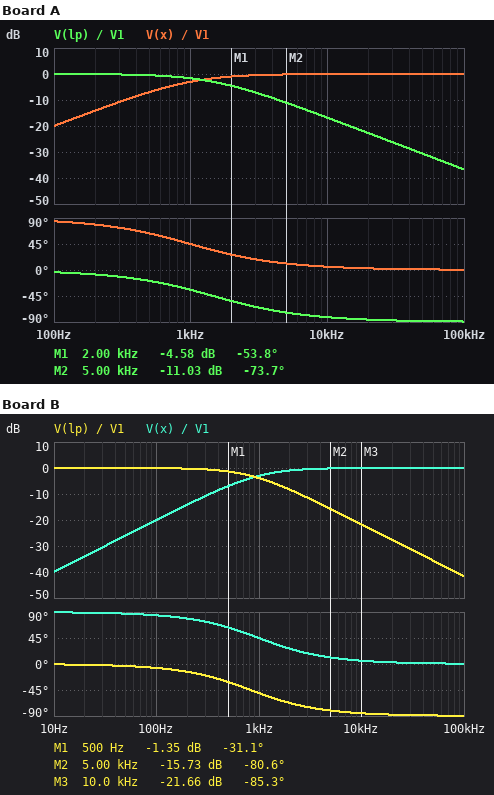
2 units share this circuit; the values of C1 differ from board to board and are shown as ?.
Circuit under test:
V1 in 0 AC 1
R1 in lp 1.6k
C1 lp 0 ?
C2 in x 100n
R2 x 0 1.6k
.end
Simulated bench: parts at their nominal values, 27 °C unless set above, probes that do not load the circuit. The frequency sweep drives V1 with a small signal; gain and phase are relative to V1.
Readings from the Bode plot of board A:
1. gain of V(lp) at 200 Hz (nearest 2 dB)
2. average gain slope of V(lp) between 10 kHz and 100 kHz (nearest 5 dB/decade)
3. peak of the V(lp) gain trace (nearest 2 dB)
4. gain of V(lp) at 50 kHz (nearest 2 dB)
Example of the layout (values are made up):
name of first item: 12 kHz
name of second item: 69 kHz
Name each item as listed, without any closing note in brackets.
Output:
gain of V(lp) at 200 Hz: 0 dB
average gain slope of V(lp) between 10 kHz and 100 kHz: -20 dB/decade
peak of the V(lp) gain trace: 0 dB
gain of V(lp) at 50 kHz: -30 dB
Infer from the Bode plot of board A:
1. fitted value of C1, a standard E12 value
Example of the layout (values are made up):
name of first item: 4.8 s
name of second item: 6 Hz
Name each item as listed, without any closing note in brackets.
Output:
fitted value of C1, a standard E12 value: 68 nF
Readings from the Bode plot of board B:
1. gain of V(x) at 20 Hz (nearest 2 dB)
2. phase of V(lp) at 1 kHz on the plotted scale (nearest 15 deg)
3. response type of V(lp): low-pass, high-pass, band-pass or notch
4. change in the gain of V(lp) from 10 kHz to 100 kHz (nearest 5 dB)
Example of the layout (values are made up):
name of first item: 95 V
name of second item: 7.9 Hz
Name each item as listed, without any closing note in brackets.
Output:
gain of V(x) at 20 Hz: -34 dB
phase of V(lp) at 1 kHz on the plotted scale: -45 deg
response type of V(lp): low-pass, high-pass, band-pass or notch: low-pass
change in the gain of V(lp) from 10 kHz to 100 kHz: -20 dB
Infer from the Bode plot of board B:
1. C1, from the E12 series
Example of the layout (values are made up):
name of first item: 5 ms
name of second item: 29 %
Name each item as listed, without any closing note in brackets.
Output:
C1, from the E12 series: 120 nF
